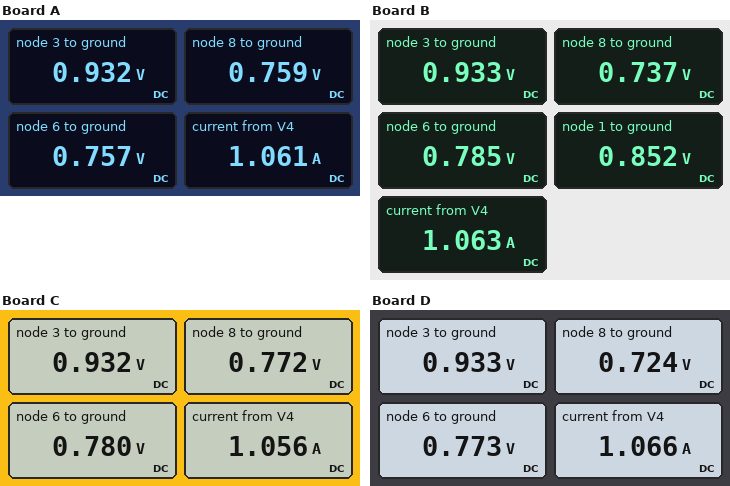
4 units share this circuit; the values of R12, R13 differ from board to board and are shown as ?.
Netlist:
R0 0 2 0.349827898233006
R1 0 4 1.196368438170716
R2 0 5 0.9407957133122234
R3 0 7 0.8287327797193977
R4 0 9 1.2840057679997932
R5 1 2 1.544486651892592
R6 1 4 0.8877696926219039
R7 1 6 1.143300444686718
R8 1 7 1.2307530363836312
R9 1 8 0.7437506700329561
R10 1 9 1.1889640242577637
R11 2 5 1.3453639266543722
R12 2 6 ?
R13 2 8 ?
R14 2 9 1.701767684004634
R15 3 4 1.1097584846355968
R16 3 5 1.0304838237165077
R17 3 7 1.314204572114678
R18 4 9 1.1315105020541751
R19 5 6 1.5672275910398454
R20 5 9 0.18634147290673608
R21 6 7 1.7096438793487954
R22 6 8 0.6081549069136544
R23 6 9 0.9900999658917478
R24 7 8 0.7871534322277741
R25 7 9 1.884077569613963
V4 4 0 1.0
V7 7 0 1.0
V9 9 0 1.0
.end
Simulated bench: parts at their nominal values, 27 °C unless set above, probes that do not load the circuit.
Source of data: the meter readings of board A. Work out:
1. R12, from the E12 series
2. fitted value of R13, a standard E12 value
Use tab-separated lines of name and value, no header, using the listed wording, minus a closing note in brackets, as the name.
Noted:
R12, from the E12 series	0.39 Ω
fitted value of R13, a standard E12 value	0.47 Ω
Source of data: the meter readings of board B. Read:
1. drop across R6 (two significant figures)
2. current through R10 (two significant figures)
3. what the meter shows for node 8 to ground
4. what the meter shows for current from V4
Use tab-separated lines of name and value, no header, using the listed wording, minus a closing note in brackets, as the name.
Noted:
drop across R6	150 mV
current through R10	120 mA
what the meter shows for node 8 to ground	0.737 V
what the meter shows for current from V4	1.063 A
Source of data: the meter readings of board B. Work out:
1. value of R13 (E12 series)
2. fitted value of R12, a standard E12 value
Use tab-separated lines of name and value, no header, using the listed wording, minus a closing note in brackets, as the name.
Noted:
value of R13	0.33 Ω
fitted value of R12, a standard E12 value	0.68 Ω
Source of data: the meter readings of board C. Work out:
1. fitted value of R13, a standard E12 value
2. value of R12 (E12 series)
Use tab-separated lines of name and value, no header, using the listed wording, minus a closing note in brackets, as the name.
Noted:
fitted value of R13, a standard E12 value	0.56 Ω
value of R12	0.56 Ω
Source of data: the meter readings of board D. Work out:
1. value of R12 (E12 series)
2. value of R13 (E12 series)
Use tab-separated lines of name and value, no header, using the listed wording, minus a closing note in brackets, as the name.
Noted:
value of R12	0.56 Ω
value of R13	0.27 Ω
